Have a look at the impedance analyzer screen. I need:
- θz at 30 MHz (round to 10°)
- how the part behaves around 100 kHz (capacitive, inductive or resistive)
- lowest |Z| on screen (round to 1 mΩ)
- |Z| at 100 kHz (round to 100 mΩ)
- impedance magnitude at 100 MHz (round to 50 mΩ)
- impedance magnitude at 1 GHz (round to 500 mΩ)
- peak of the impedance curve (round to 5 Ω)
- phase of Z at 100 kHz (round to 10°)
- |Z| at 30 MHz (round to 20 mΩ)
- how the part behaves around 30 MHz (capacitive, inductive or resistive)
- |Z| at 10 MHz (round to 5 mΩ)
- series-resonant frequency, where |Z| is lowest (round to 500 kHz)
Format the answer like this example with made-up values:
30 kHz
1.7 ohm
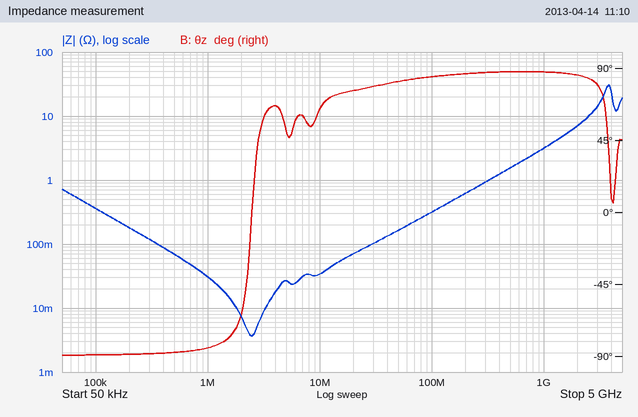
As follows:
80°
capacitive
4 mΩ
400 mΩ
300 mΩ
3.0 Ω
30 Ω
-90°
100 mΩ
inductive
35 mΩ
2.5 MHz
